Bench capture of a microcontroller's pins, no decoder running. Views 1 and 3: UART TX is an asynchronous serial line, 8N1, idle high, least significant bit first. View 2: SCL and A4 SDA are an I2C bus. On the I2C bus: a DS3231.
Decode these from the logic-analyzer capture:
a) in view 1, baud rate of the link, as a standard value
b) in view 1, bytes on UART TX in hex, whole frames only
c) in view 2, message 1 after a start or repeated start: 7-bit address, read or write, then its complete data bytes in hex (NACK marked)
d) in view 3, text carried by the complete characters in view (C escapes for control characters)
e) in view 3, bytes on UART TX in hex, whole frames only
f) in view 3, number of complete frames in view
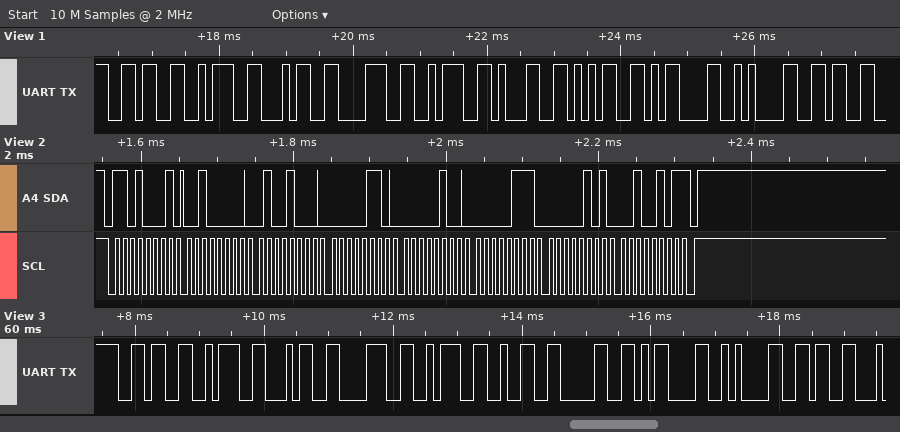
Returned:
9600 baud
36 3A 34 38 3A 31 35 0D 0A 36
0x68 read: 20 48 06 04 07 05 25 NACK
"6:48:20\r\n6"
36 3A 34 38 3A 32 30 0D 0A 36
10
